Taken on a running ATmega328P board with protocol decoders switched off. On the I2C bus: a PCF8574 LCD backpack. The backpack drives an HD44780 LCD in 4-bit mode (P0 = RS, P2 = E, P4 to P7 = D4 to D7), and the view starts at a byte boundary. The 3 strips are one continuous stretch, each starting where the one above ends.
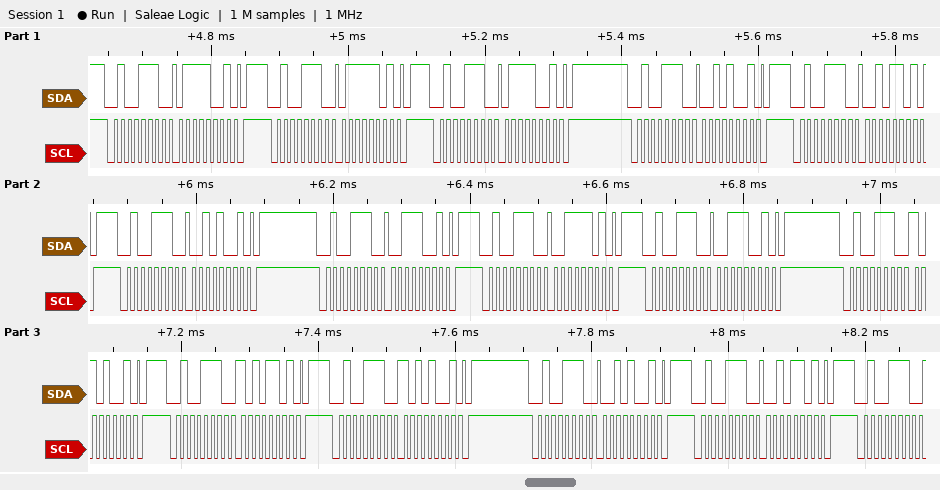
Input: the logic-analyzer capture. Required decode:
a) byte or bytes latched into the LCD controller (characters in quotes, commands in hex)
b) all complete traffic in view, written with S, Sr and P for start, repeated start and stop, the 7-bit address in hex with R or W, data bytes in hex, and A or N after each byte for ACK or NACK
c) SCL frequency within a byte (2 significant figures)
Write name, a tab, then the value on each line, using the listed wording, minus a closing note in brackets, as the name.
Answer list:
byte or bytes latched into the LCD controller	'r' ':'
all complete traffic in view, written with S, Sr and P for start, repeated start and stop, the 7-bit address in hex with R or W, data bytes in hex, and A or N after each byte for ACK or NACK	S 27W A 79 A P S 27W A 7D A P S 27W A 79 A P S 27W A 29 A P S 27W A 2D A P S 27W A 29 A P S 27W A 39 A P S 27W A 3D A P S 27W A 39 A P S 27W A A9 A P S 27W A AD A P S 27W A A9 A P S 27W A 29 A P S 27W A 2D A P S 27W A
SCL frequency within a byte	100 kHz
